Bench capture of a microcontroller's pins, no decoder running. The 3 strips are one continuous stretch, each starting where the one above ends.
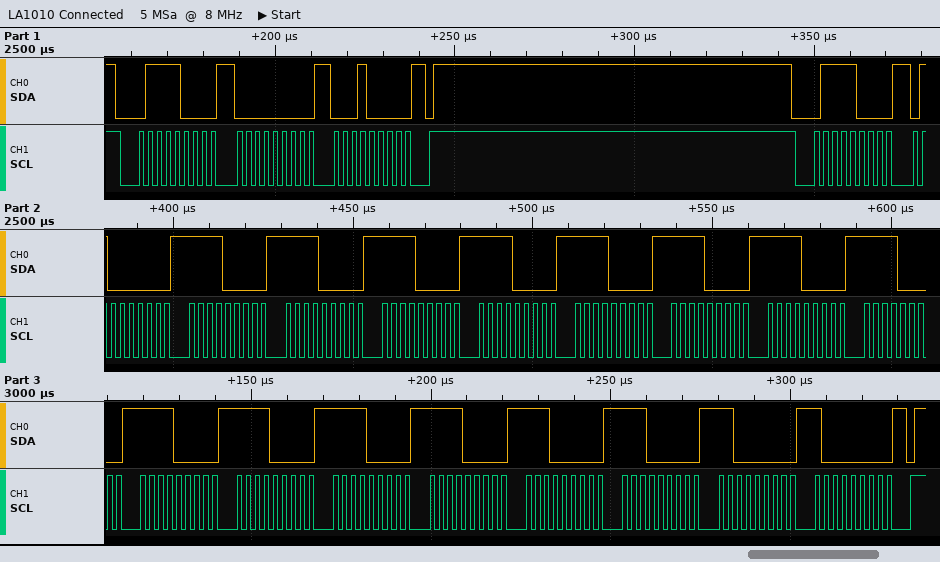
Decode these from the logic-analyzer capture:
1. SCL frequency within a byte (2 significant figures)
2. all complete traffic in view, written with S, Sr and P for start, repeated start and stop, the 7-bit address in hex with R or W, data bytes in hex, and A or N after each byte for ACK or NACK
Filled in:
400 kHz
S 3CW A 00 A 10 A P S 3CW A 40 A F0 A F0 A F0 A F0 A F0 A F0 A F0 A F0 A F0 A F0 A F0 A F0 A E0 A E0 A C0 A 80 A P
